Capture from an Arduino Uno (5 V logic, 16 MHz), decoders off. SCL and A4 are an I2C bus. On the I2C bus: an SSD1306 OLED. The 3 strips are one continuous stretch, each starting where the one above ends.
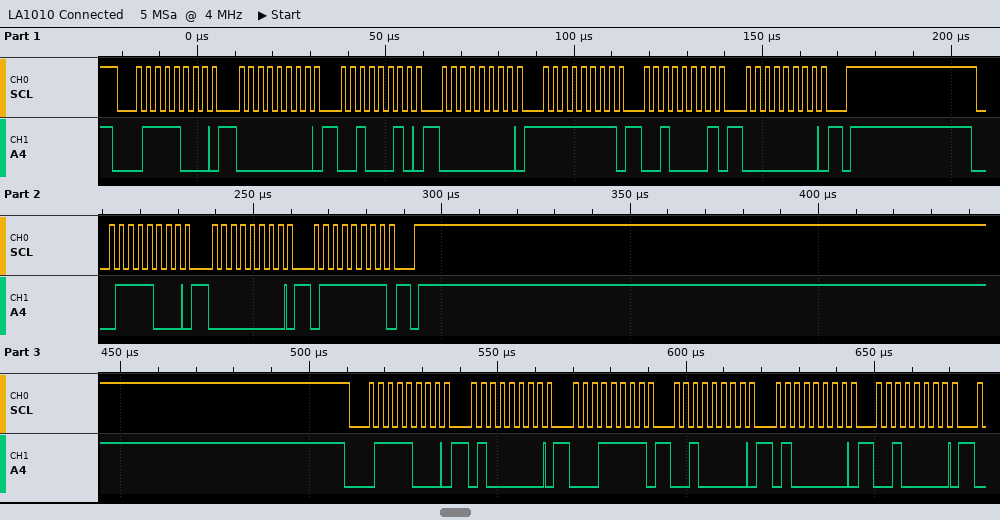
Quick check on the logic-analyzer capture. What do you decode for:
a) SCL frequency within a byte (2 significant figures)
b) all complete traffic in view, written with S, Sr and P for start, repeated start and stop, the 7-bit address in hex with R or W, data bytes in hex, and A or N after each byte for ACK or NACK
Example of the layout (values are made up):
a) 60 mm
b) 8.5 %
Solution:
a) 400 kHz
b) S 3CW A 00 A 22 A 00 A FF A 21 A 00 A P S 3CW A 00 A 7F A P S 3CW A 40 A 1F A 20 A 40 A 20 A
